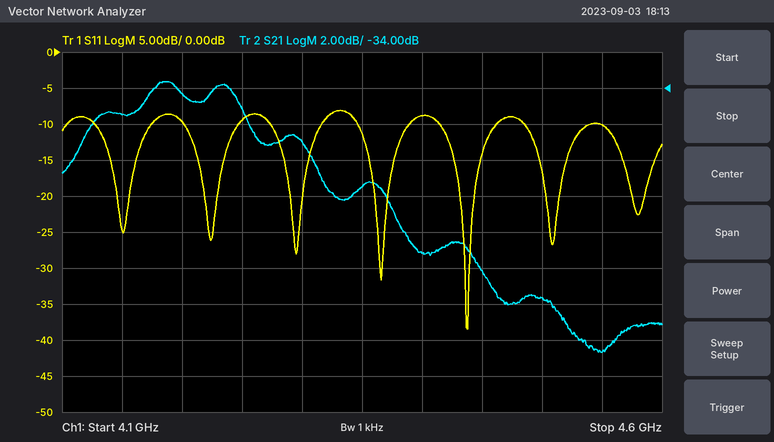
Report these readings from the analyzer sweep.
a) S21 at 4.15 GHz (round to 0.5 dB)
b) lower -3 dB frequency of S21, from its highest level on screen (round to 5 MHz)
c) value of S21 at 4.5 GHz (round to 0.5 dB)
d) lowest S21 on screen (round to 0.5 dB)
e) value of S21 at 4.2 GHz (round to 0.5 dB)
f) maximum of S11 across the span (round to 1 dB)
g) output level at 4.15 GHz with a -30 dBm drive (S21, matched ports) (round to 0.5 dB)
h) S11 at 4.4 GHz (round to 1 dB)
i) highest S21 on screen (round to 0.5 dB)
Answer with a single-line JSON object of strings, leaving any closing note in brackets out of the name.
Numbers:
{"S21 at 4.15 GHz": "-35.5 dB", "lower -3 dB frequency of S21, from its highest level on screen": "4.120 GHz", "value of S21 at 4.5 GHz": "-45.5 dB", "lowest S21 on screen": "-48.5 dB", "value of S21 at 4.2 GHz": "-34.5 dB", "maximum of S11 across the span": "-8 dB", "output level at 4.15 GHz with a -30 dBm drive (S21, matched ports)": "-65.5 dBm", "S11 at 4.4 GHz": "-9 dB", "highest S21 on screen": "-33.5 dB"}
